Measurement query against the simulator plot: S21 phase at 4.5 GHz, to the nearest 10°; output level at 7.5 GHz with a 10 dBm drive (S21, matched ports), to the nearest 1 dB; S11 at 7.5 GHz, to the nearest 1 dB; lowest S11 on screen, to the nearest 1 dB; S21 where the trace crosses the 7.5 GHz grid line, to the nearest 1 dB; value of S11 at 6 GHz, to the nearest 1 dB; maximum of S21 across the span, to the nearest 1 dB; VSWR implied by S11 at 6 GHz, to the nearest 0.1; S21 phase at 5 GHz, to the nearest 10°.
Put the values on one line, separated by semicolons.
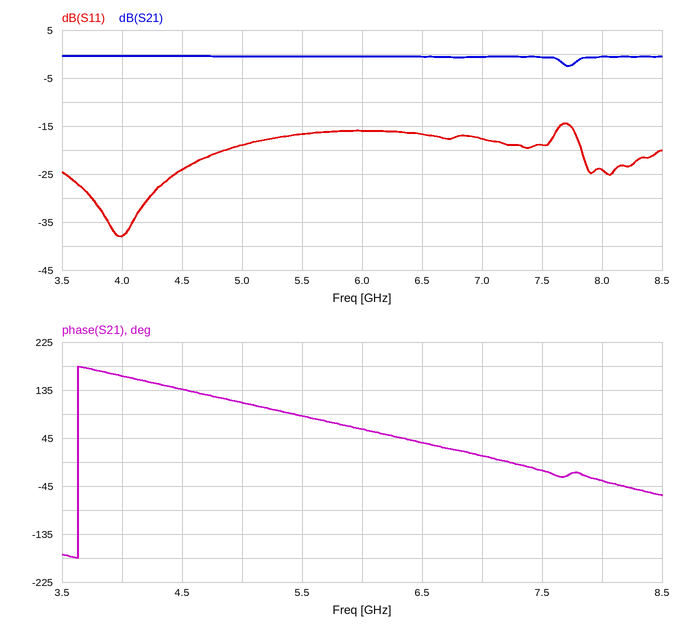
140°; 9 dBm; -19 dB; -38 dB; -1 dB; -16 dB; 0 dB; 1.4; 110°
